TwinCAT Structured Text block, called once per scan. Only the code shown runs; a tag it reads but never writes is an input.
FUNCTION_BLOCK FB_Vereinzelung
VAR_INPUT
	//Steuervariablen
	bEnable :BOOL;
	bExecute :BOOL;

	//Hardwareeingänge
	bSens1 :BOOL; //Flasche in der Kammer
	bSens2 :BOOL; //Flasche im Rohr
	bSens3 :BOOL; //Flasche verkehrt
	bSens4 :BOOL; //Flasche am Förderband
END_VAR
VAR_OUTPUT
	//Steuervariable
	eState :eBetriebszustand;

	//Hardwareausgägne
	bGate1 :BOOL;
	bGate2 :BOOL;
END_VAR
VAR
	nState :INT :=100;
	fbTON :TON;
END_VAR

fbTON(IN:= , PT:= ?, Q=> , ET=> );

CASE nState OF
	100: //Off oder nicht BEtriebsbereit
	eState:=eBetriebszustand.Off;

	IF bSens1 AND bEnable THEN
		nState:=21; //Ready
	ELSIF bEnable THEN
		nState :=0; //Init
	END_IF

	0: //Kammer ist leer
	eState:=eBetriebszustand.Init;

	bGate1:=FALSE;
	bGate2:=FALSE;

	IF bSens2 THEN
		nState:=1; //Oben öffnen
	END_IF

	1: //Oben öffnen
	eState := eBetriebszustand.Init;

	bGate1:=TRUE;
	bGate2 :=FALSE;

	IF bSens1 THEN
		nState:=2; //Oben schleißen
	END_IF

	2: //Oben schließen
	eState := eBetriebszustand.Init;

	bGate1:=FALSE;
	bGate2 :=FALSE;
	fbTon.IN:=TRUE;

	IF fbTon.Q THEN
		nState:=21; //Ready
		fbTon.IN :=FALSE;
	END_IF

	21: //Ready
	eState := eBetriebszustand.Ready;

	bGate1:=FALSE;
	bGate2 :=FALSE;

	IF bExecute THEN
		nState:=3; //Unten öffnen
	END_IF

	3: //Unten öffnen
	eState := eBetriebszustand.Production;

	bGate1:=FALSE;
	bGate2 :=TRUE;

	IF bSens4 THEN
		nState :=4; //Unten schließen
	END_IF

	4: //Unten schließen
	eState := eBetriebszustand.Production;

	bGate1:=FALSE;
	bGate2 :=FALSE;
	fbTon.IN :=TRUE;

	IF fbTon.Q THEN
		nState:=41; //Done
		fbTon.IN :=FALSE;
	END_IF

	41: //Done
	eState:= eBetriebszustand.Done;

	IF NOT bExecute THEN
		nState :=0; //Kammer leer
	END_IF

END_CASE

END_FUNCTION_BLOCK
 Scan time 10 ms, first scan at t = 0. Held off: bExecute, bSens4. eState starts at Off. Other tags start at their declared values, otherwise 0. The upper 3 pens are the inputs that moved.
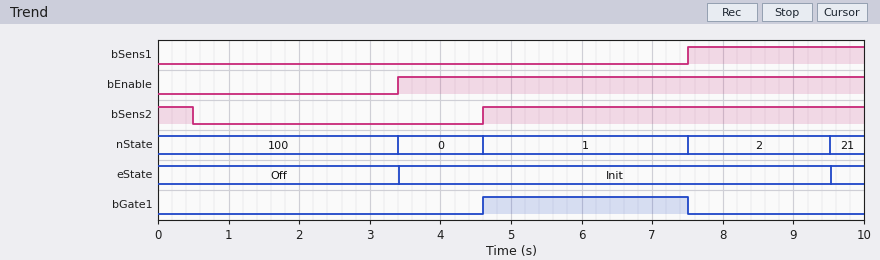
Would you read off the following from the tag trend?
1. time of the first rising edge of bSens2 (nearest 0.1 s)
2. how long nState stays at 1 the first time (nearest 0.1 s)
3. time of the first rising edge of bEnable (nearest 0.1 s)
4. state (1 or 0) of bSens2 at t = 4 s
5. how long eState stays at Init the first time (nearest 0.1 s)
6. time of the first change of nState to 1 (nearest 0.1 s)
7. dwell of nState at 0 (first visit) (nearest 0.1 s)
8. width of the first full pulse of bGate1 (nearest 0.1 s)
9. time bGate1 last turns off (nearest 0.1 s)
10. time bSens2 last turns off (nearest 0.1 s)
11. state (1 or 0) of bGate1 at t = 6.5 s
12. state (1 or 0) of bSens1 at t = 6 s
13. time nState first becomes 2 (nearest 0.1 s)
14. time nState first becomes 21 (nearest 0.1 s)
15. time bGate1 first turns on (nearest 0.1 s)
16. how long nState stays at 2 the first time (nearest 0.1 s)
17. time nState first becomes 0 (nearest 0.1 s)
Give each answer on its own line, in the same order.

4.6 s
2.9 s
3.4 s
0
6.1 s
4.6 s
1.2 s
2.9 s
7.5 s
0.5 s
1
0
7.5 s
9.5 s
4.6 s
2.0 s
3.4 s
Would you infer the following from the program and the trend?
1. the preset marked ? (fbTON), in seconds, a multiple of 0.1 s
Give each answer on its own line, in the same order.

2.0 s
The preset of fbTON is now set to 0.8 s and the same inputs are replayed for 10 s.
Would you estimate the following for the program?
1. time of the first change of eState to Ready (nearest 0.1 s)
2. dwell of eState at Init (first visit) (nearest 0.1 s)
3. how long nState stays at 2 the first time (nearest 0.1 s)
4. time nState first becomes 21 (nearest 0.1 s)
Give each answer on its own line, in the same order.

8.3 s
4.9 s
0.8 s
8.3 s
